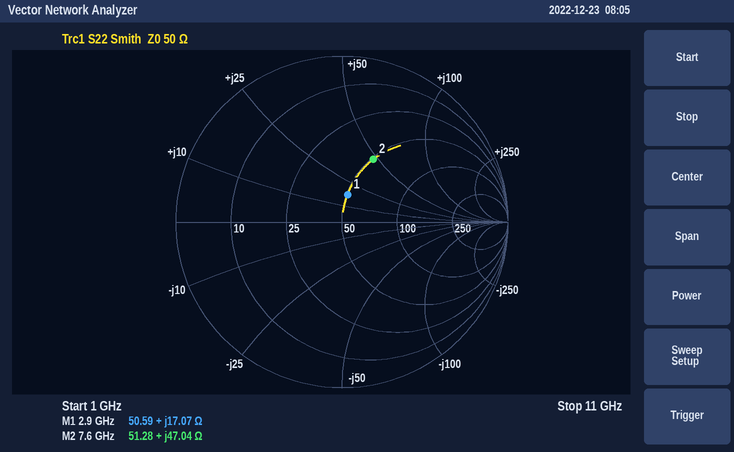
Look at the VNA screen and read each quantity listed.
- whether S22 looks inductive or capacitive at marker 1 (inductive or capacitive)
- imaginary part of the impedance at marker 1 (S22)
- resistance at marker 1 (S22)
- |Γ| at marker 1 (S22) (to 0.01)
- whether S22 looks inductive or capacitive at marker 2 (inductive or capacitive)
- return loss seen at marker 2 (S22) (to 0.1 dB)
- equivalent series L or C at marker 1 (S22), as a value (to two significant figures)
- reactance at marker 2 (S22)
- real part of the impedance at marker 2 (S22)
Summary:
inductive
+17.07 Ω
50.59 Ω
0.17
inductive
7.5 dB
940 pH
+47.04 Ω
51.28 Ω
